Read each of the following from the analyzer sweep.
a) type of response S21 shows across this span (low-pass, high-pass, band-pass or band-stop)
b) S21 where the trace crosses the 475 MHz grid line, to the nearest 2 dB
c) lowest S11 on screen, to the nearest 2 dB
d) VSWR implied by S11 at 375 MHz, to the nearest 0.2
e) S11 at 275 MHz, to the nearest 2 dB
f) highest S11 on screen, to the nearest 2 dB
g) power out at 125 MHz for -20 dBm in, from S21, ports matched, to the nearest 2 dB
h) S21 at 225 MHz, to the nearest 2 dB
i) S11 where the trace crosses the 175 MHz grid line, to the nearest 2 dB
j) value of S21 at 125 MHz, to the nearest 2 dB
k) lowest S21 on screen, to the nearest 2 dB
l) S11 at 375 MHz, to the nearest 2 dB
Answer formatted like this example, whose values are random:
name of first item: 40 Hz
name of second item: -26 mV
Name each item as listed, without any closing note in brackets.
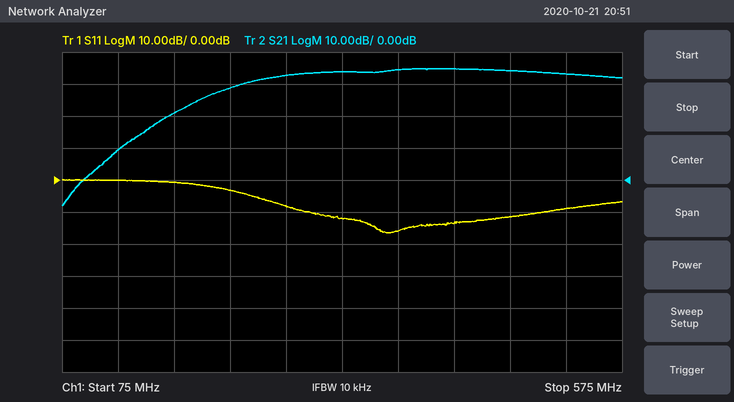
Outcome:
type of response S21 shows across this span: high-pass
S21 where the trace crosses the 475 MHz grid line, to the nearest 2 dB: 34 dB
lowest S11 on screen, to the nearest 2 dB: -16 dB
VSWR implied by S11 at 375 MHz, to the nearest 0.2: 1.4
S11 at 275 MHz, to the nearest 2 dB: -8 dB
highest S11 on screen, to the nearest 2 dB: 0 dB
power out at 125 MHz for -20 dBm in, from S21, ports matched, to the nearest 2 dB: -10 dBm
S21 at 225 MHz, to the nearest 2 dB: 28 dB
S11 where the trace crosses the 175 MHz grid line, to the nearest 2 dB: 0 dB
value of S21 at 125 MHz, to the nearest 2 dB: 10 dB
lowest S21 on screen, to the nearest 2 dB: -8 dB
S11 at 375 MHz, to the nearest 2 dB: -16 dB
